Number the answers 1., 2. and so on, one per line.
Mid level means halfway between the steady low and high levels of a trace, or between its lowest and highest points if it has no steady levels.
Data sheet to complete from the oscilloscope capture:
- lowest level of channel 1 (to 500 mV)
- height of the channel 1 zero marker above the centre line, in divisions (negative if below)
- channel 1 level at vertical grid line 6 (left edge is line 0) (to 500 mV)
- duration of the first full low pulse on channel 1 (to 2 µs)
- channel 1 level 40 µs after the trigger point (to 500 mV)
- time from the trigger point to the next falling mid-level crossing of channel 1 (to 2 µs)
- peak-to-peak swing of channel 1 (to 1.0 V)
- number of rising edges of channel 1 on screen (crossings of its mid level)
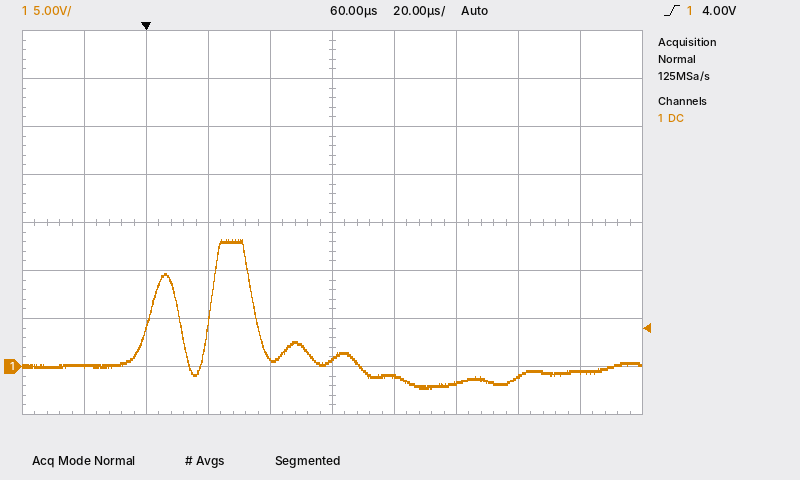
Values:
1. -2.5 V
2. -3.0 div
3. -1.0 V
4. 10 µs
5. 1.0 V
6. 10 µs
7. 16.0 V
8. 2
